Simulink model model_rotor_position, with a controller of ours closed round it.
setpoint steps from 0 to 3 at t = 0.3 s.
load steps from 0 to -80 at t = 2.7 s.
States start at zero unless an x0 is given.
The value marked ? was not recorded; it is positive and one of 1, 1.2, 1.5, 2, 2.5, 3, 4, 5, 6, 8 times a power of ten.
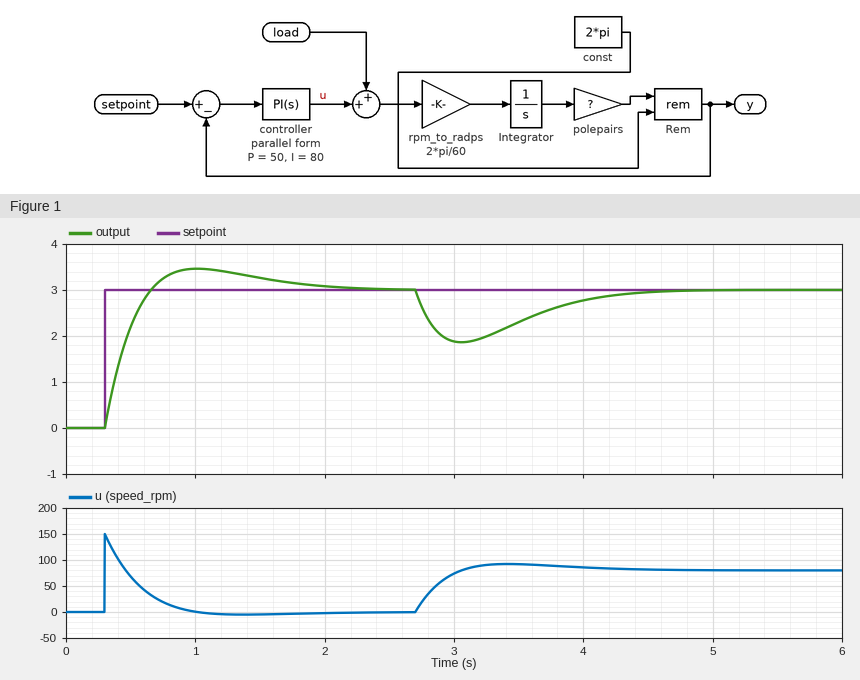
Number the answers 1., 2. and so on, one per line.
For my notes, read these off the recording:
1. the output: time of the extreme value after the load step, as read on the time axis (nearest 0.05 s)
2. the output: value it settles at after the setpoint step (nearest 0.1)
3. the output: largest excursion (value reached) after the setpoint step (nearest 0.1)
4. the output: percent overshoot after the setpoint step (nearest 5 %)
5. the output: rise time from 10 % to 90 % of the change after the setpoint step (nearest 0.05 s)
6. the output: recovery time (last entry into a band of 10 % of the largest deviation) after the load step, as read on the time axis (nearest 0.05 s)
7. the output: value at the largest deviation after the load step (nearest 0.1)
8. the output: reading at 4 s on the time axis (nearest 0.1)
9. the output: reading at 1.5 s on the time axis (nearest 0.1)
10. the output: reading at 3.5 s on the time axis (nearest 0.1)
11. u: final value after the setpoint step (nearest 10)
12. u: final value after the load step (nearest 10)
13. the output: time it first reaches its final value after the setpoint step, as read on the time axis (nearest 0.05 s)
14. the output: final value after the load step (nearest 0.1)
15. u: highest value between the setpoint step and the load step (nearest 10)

1. 3.05 s
2. 3.0
3. 3.5
4. 15 %
5. 0.25 s
6. 4.25 s
7. 1.9
8. 2.8
9. 3.3
10. 2.3
11. 0
12. 80
13. 0.65 s
14. 3.0
15. 150
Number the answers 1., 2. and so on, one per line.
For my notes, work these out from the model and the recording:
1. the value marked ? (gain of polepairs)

1. 1
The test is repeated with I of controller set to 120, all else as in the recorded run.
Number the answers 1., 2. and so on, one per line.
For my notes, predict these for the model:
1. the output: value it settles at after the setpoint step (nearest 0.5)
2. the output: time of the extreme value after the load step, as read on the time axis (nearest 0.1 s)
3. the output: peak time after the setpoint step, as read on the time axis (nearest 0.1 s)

1. 3.0
2. 3.0 s
3. 0.9 s
